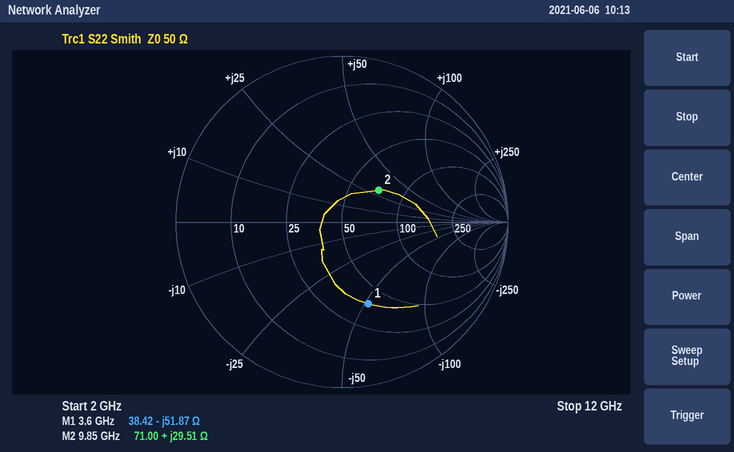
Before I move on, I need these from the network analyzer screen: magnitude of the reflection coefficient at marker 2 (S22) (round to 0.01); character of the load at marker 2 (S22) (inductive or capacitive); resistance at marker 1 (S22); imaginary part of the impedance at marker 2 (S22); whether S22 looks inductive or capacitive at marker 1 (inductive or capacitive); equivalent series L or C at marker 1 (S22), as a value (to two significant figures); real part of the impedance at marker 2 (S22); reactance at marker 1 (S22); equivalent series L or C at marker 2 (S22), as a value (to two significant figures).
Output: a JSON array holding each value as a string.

["0.29", "inductive", "38.42 Ω", "+29.51 Ω", "capacitive", "850 fF", "71.00 Ω", "-51.87 Ω", "480 pH"]
